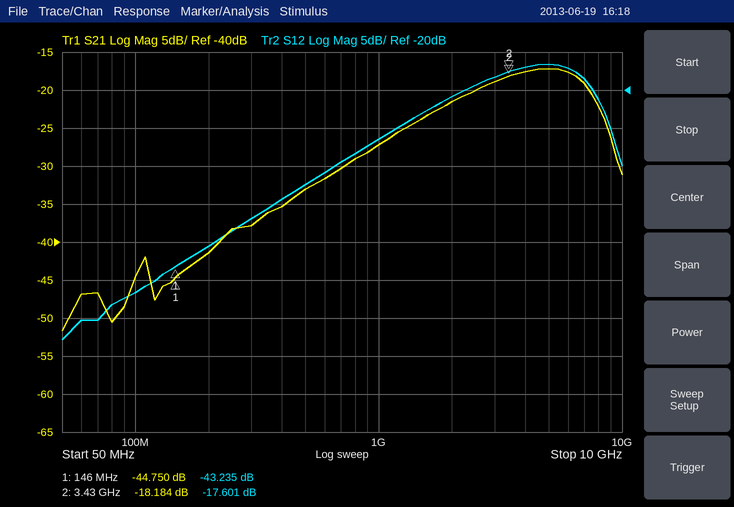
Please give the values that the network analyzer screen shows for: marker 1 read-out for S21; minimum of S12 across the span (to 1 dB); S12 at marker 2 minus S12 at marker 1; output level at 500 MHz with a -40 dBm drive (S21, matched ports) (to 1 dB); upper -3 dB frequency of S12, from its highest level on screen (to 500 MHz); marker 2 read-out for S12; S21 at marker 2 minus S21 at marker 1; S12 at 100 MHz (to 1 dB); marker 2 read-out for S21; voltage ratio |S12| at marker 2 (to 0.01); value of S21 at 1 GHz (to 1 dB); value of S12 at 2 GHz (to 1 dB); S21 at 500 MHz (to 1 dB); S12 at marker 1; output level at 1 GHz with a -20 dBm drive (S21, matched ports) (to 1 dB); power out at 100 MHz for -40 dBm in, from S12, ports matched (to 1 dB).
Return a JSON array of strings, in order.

["-44.750 dB", "-53 dB", "25.634 dB", "-73 dBm", "7.5 GHz", "-17.601 dB", "26.566 dB", "-47 dB", "-18.184 dB", "0.13", "-27 dB", "-21 dB", "-33 dB", "-43.235 dB", "-47 dBm", "-87 dBm"]
